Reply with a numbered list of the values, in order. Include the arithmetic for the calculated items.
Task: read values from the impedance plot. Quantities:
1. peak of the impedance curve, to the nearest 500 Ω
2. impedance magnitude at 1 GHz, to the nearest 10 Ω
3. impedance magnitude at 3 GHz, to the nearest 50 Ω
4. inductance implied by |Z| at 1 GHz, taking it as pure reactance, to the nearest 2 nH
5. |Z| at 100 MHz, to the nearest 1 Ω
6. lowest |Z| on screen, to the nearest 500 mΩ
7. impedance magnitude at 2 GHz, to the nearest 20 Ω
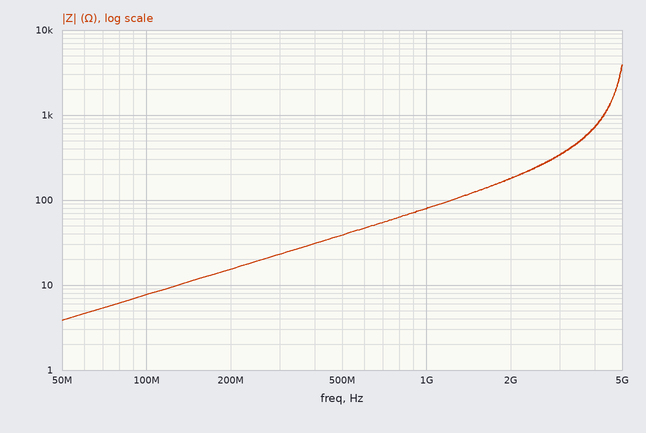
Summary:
1. 4.0 kΩ
2. 80 Ω
3. 350 Ω
4. L = 80 Ω/(2π × 1 GHz) ≈ 12.7 nH, so 12 nH to the nearest 2 nH
5. 8 Ω
6. 4.0 Ω
7. 180 Ω
